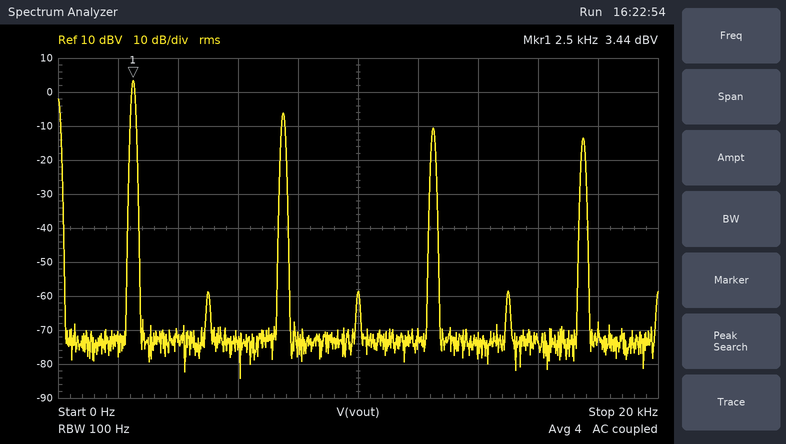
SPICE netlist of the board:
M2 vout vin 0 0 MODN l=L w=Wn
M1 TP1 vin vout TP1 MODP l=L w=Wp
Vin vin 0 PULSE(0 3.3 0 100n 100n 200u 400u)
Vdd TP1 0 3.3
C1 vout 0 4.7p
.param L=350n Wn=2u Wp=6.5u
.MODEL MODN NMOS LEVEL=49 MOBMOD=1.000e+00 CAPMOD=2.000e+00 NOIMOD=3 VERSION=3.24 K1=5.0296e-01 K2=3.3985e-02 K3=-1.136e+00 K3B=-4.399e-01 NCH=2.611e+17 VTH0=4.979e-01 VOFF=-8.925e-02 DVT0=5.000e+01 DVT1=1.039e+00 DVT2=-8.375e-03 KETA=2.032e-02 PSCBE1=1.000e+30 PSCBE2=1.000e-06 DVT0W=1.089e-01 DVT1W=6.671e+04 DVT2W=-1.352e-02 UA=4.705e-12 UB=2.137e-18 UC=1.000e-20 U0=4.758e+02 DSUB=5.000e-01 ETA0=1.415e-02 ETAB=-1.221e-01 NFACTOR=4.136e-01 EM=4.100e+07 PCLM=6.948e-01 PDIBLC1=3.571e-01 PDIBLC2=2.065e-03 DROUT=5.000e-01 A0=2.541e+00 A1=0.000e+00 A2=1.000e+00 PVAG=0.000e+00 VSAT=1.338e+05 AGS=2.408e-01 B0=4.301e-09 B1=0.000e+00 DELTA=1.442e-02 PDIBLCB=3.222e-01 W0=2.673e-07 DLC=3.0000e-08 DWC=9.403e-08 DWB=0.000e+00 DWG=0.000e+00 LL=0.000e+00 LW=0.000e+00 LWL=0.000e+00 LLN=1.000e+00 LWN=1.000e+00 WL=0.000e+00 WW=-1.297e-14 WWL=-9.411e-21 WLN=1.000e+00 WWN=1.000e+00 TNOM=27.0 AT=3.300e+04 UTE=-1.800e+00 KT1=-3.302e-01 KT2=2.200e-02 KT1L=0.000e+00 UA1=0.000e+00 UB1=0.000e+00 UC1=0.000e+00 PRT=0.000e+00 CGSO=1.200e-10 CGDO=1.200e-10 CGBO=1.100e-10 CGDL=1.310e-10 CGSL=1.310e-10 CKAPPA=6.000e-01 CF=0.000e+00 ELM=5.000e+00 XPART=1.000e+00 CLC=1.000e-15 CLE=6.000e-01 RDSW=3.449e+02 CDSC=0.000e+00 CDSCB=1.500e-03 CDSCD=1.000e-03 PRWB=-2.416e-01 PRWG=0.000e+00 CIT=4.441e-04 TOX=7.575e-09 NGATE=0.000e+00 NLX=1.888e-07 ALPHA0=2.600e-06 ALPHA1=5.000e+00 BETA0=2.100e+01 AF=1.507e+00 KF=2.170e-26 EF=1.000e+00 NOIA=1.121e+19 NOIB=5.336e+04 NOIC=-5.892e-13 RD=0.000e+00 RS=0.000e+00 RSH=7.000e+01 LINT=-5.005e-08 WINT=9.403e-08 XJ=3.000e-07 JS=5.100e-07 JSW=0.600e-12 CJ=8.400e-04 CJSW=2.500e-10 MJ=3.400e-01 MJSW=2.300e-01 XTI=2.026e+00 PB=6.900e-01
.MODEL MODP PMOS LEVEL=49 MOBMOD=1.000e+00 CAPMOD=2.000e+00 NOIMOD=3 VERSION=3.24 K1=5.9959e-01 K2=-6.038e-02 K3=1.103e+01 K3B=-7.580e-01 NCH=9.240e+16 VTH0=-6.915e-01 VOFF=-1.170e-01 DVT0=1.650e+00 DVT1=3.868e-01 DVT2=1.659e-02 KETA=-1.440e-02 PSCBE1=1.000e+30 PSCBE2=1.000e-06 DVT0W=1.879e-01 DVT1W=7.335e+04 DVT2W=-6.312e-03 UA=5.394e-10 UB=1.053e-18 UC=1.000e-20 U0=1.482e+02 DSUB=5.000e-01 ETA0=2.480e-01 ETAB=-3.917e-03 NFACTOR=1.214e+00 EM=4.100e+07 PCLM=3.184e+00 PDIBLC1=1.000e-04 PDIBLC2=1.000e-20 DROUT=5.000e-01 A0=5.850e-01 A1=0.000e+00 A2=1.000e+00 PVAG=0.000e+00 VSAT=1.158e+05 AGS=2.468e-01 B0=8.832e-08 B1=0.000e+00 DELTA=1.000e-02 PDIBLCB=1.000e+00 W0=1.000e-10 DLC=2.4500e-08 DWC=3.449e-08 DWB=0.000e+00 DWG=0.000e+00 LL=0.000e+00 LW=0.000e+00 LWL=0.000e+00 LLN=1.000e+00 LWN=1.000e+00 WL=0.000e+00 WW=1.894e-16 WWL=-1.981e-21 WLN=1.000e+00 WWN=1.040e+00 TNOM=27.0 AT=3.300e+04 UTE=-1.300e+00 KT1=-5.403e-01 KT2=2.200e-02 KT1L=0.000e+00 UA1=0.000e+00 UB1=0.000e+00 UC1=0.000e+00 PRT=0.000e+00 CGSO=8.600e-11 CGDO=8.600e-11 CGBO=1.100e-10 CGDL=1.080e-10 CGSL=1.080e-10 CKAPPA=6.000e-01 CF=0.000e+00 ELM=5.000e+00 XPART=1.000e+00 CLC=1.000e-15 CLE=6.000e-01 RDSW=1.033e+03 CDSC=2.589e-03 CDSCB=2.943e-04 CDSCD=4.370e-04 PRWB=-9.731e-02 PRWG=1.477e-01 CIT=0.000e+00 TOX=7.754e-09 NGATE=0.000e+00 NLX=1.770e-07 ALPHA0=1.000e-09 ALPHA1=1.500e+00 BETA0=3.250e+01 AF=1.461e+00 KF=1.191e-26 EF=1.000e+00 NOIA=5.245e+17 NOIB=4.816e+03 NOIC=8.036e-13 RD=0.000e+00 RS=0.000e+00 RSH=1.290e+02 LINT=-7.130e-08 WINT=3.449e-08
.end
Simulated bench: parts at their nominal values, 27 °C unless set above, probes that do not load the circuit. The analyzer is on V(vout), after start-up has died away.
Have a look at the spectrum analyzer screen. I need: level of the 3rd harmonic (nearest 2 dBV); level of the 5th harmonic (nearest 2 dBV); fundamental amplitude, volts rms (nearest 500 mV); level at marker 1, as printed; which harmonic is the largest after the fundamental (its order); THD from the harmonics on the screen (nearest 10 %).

-6 dBV
-10 dBV
1.5 V
3.44 dBV
3
40 %
